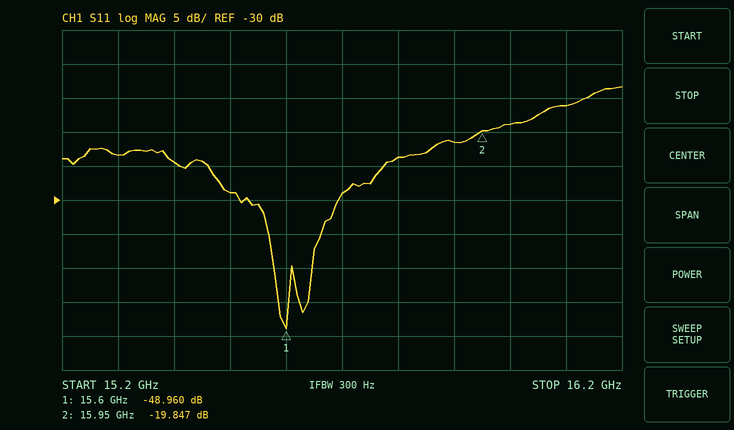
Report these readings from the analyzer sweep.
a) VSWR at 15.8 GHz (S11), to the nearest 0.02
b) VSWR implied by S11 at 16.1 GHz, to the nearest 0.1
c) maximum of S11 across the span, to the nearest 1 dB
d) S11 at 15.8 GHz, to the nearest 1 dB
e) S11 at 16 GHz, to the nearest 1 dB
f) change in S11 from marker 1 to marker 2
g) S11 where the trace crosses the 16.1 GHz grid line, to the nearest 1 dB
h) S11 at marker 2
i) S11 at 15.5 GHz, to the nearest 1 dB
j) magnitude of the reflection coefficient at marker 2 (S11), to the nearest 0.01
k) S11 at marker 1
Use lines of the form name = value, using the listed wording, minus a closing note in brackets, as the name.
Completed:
VSWR at 15.8 GHz (S11), to the nearest 0.02 = 1.14
VSWR implied by S11 at 16.1 GHz, to the nearest 0.1 = 1.4
maximum of S11 across the span, to the nearest 1 dB = -13 dB
S11 at 15.8 GHz, to the nearest 1 dB = -24 dB
S11 at 16 GHz, to the nearest 1 dB = -19 dB
change in S11 from marker 1 to marker 2 = 29.113 dB
S11 where the trace crosses the 16.1 GHz grid line, to the nearest 1 dB = -16 dB
S11 at marker 2 = -19.847 dB
S11 at 15.5 GHz, to the nearest 1 dB = -29 dB
magnitude of the reflection coefficient at marker 2 (S11), to the nearest 0.01 = 0.10
S11 at marker 1 = -48.960 dB
